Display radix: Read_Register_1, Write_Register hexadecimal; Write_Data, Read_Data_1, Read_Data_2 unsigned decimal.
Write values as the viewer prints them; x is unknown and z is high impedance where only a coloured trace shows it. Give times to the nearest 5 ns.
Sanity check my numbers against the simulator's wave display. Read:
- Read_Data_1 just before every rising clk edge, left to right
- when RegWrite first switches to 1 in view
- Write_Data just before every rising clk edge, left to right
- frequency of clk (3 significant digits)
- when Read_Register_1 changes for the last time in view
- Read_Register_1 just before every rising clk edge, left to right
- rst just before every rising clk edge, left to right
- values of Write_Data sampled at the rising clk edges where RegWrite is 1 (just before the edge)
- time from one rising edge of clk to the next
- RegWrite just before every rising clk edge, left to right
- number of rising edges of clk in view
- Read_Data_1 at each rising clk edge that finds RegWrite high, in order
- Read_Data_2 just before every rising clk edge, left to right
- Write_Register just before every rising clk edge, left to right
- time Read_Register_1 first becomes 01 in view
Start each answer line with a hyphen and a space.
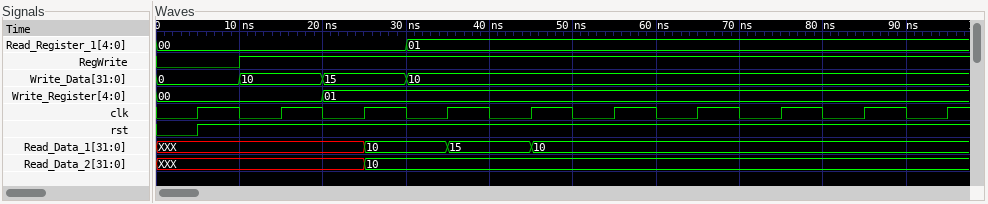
- XXX, XXX, XXX, 10, 15, 10, 10, 10, 10, 10
- 10 ns
- 0, 10, 15, 10, 10, 10, 10, 10, 10, 10
- 100 MHz
- 30 ns
- 00, 00, 00, 01, 01, 01, 01, 01, 01, 01
- 0 1 1 1 1 1 1 1 1 1
- 10, 15, 10, 10, 10, 10, 10, 10, 10
- 10 ns
- 0 1 1 1 1 1 1 1 1 1
- 10
- XXX, XXX, 10, 15, 10, 10, 10, 10, 10
- XXX, XXX, XXX, 10, 10, 10, 10, 10, 10, 10
- 00, 00, 01, 01, 01, 01, 01, 01, 01, 01
- 30 ns
